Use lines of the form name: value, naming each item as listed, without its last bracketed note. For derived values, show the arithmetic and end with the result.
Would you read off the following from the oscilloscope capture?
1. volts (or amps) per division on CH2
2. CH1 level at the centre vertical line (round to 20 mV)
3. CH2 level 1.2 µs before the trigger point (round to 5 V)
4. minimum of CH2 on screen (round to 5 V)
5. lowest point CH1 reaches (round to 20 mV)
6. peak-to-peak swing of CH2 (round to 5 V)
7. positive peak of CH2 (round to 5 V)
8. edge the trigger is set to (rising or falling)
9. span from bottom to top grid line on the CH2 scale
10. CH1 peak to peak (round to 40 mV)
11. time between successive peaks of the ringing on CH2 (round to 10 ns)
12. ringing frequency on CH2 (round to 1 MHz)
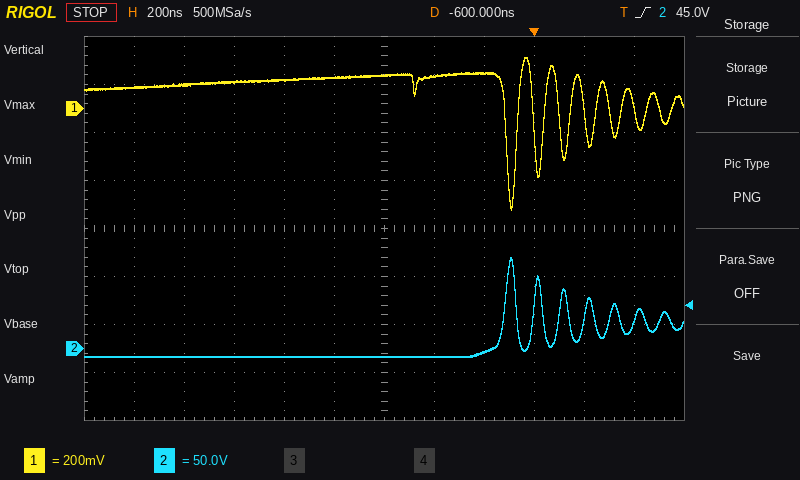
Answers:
volts (or amps) per division on CH2: 50 V
CH1 level at the centre vertical line: 140 mV
CH2 level 1.2 µs before the trigger point: -10 V
minimum of CH2 on screen: -10 V
lowest point CH1 reaches: -420 mV
peak-to-peak swing of CH2: 95 V − (-10 V) = 105 V
positive peak of CH2: 95 V
edge the trigger is set to: rising
span from bottom to top grid line on the CH2 scale: 400 V
CH1 peak to peak: 640 mV
time between successive peaks of the ringing on CH2: 100 ns
ringing frequency on CH2: 1 / 100 ns ≈ 10 MHz
